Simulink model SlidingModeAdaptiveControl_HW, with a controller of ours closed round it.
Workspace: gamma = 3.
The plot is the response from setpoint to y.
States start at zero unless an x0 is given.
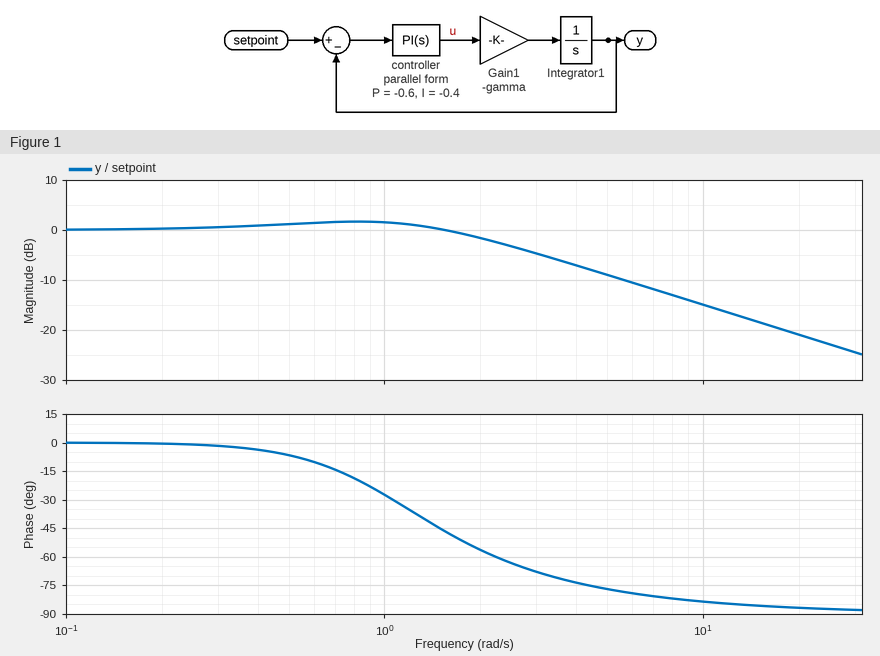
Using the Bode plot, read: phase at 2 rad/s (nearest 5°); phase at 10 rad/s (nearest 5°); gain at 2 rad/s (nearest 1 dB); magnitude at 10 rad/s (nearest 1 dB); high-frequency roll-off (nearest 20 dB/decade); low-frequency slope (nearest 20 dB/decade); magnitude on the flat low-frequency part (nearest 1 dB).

-55°
-85°
-2 dB
-15 dB
-20 dB/decade
0 dB/decade
0 dB
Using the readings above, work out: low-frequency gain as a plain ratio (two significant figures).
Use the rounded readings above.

1.0
